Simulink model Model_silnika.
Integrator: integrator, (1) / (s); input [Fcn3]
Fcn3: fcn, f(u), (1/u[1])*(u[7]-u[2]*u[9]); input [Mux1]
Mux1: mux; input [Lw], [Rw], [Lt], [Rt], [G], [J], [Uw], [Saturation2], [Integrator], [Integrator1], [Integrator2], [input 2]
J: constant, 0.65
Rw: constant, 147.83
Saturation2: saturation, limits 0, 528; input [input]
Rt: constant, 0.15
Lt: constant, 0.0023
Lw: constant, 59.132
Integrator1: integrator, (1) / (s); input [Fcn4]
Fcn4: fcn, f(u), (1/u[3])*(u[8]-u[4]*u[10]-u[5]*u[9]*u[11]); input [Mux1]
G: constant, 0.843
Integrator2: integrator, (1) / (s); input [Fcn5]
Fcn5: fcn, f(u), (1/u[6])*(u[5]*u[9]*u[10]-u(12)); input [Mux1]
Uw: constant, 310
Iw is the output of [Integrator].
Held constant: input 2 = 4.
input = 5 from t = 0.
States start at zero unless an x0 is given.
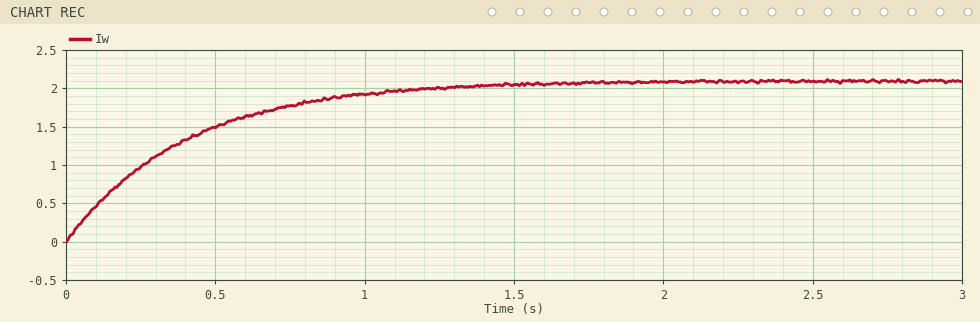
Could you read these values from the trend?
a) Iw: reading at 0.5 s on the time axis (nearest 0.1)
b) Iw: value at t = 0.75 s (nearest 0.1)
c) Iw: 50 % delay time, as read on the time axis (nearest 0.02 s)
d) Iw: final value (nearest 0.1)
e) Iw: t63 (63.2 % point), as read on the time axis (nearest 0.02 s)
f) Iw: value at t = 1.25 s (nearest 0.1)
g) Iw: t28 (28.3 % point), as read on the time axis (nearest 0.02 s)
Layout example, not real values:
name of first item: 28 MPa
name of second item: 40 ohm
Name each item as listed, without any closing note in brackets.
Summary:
Iw: reading at 0.5 s on the time axis: 1.5
Iw: value at t = 0.75 s: 1.8
Iw: 50 % delay time, as read on the time axis: 0.28 s
Iw: final value: 2.1
Iw: t63 (63.2 % point), as read on the time axis: 0.40 s
Iw: value at t = 1.25 s: 2.0
Iw: t28 (28.3 % point), as read on the time axis: 0.14 s
